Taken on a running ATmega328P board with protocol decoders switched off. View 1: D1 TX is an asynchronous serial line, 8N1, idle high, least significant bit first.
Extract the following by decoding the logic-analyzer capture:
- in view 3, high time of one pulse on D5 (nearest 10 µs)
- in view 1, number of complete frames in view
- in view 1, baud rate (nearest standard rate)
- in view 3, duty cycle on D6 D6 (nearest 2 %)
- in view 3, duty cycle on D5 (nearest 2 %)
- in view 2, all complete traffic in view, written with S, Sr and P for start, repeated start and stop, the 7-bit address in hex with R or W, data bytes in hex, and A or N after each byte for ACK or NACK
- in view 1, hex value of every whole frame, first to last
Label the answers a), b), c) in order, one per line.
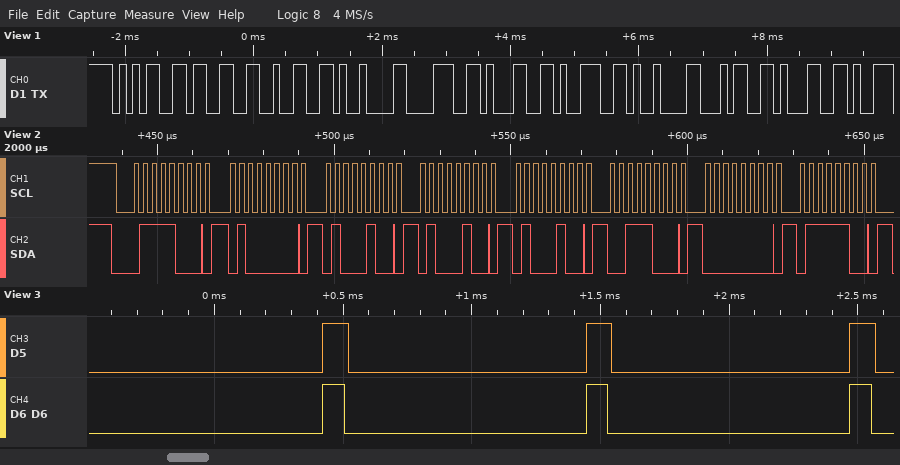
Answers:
a) 100 µs
b) 10
c) 9600 baud
d) 8 %
e) 10 %
f) S 3CW A 40 A 44 A 44 A 44 A 38 A 00 A 7C A
g) 35 33 32 09 38 31 39 09 34 31
